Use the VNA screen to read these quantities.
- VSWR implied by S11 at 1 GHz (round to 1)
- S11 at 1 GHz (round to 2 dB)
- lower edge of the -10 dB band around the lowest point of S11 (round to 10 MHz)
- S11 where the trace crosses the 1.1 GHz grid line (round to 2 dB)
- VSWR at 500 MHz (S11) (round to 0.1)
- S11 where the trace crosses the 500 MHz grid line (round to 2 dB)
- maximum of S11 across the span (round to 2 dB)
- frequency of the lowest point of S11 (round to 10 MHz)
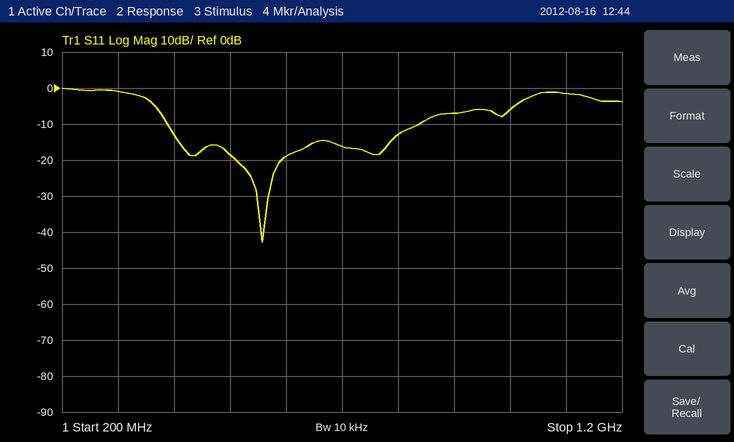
3
-6 dB
390 MHz
-2 dB
1.3
-18 dB
0 dB
560 MHz
